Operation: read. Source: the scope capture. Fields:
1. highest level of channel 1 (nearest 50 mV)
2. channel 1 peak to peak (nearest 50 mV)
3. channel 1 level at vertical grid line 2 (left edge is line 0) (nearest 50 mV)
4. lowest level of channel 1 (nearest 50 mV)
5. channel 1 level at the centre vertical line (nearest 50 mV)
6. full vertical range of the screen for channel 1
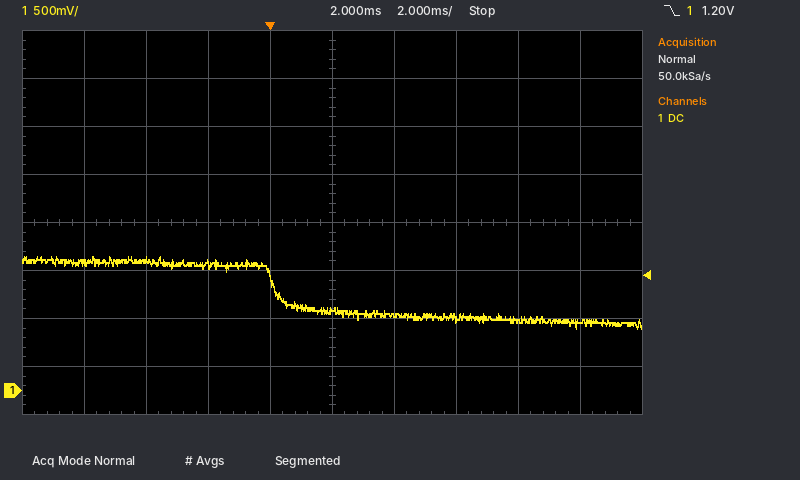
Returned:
1.40 V
750 mV
1.35 V
650 mV
850 mV
4 V
